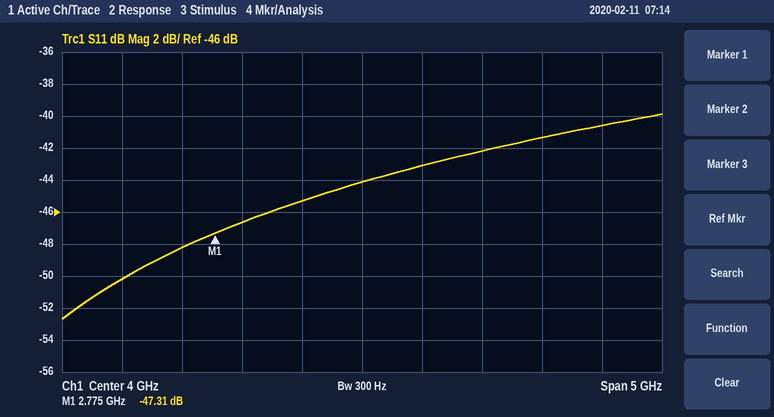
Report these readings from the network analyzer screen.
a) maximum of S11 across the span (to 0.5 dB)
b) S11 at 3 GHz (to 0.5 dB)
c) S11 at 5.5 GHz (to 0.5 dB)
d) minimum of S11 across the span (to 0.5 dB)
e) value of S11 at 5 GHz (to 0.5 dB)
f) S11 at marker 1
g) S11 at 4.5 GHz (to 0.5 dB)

-40.0 dB
-46.5 dB
-41.5 dB
-52.5 dB
-42.0 dB
-47.31 dB
-43.0 dB
